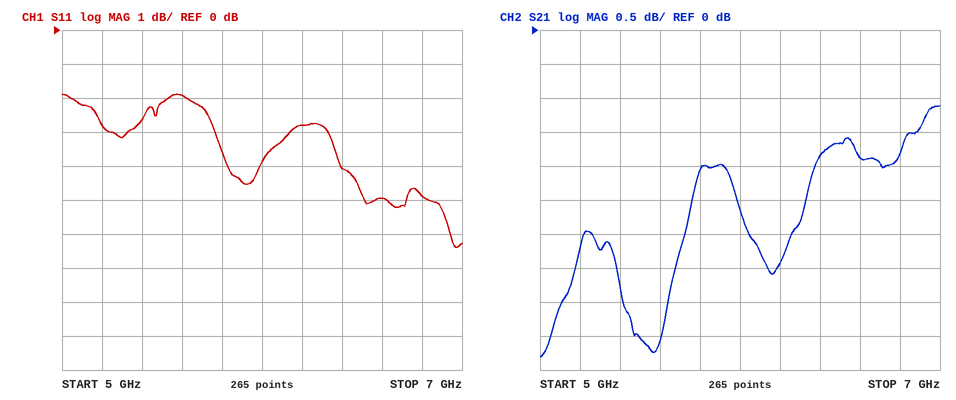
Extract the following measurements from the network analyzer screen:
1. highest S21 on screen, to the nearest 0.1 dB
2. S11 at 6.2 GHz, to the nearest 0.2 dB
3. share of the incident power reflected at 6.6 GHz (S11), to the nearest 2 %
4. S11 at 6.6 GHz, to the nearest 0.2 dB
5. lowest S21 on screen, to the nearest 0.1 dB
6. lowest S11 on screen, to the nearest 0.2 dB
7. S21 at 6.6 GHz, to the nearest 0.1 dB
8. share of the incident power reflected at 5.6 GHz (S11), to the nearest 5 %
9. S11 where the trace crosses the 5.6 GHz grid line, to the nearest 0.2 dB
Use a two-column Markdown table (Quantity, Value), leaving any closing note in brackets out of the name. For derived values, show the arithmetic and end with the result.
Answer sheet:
| Quantity | Value |
|---|---|
| highest S21 on screen, to the nearest 0.1 dB | -1.1 dB |
| S11 at 6.2 GHz, to the nearest 0.2 dB | -2.8 dB |
| share of the incident power reflected at 6.6 GHz (S11), to the nearest 2 % | 10^(-5/10) ≈ 32 % |
| S11 at 6.6 GHz, to the nearest 0.2 dB | -5.0 dB |
| lowest S21 on screen, to the nearest 0.1 dB | -4.8 dB |
| lowest S11 on screen, to the nearest 0.2 dB | -6.4 dB |
| S21 at 6.6 GHz, to the nearest 0.1 dB | -1.9 dB |
| share of the incident power reflected at 5.6 GHz (S11), to the nearest 5 % | 10^(-2/10) ≈ 63.1 %, so 65 % to the nearest 5 % |
| S11 where the trace crosses the 5.6 GHz grid line, to the nearest 0.2 dB | -2.0 dB |
